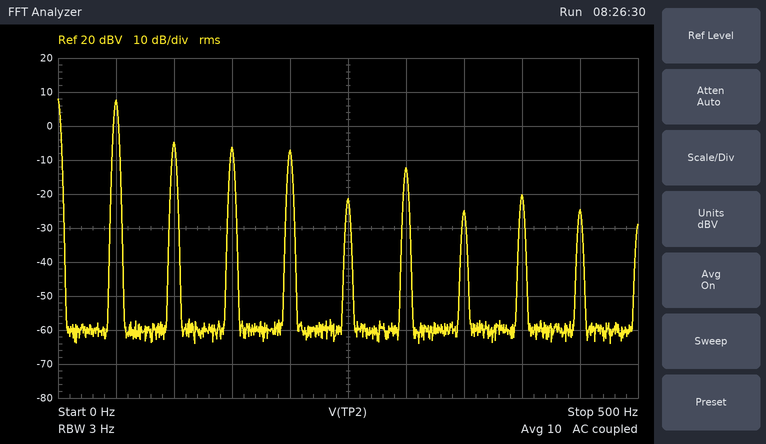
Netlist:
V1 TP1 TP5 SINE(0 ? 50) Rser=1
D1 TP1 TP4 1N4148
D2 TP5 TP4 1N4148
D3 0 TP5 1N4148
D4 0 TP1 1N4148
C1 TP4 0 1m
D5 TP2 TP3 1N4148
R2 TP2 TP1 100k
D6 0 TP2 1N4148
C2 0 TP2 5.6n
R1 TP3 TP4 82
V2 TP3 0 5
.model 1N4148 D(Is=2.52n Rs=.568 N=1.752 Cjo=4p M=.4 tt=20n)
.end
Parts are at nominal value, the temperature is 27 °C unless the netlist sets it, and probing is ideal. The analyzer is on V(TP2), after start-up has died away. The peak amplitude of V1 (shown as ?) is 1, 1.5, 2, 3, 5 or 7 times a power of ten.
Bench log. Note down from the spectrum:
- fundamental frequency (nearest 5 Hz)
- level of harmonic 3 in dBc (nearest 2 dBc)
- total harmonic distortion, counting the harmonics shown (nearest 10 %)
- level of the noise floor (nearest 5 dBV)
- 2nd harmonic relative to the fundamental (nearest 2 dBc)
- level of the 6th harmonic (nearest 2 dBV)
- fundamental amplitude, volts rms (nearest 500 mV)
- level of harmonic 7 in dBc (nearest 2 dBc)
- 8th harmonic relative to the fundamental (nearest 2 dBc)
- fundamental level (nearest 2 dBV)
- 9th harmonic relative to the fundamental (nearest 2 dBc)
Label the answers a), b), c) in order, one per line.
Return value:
a) 50 Hz
b) -14 dBc
c) 40 %
d) -60 dBV
e) -12 dBc
f) -12 dBV
g) 2.5 V
h) -32 dBc
i) -28 dBc
j) 8 dBV
k) -32 dBc
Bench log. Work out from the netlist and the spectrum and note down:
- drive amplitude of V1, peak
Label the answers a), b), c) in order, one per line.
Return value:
a) 15 V
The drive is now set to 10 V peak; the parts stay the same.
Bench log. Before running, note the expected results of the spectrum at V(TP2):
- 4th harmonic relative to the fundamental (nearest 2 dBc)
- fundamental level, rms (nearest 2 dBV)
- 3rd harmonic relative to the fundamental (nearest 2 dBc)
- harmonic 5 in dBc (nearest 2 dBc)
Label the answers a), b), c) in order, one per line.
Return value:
a) -20 dBc
b) 8 dBV
c) -12 dBc
d) -22 dBc
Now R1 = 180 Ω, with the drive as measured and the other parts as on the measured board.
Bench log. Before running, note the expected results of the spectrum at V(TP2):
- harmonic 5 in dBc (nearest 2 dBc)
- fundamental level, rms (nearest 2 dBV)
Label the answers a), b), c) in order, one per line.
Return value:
a) -34 dBc
b) 8 dBV
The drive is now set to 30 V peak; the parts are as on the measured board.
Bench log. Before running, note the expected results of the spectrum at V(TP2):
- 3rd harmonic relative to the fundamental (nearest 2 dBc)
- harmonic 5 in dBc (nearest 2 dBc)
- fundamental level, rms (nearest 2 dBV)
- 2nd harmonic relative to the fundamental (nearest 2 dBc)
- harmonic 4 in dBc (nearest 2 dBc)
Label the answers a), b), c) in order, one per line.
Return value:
a) -18 dBc
b) -24 dBc
c) 8 dBV
d) -10 dBc
e) -12 dBc
